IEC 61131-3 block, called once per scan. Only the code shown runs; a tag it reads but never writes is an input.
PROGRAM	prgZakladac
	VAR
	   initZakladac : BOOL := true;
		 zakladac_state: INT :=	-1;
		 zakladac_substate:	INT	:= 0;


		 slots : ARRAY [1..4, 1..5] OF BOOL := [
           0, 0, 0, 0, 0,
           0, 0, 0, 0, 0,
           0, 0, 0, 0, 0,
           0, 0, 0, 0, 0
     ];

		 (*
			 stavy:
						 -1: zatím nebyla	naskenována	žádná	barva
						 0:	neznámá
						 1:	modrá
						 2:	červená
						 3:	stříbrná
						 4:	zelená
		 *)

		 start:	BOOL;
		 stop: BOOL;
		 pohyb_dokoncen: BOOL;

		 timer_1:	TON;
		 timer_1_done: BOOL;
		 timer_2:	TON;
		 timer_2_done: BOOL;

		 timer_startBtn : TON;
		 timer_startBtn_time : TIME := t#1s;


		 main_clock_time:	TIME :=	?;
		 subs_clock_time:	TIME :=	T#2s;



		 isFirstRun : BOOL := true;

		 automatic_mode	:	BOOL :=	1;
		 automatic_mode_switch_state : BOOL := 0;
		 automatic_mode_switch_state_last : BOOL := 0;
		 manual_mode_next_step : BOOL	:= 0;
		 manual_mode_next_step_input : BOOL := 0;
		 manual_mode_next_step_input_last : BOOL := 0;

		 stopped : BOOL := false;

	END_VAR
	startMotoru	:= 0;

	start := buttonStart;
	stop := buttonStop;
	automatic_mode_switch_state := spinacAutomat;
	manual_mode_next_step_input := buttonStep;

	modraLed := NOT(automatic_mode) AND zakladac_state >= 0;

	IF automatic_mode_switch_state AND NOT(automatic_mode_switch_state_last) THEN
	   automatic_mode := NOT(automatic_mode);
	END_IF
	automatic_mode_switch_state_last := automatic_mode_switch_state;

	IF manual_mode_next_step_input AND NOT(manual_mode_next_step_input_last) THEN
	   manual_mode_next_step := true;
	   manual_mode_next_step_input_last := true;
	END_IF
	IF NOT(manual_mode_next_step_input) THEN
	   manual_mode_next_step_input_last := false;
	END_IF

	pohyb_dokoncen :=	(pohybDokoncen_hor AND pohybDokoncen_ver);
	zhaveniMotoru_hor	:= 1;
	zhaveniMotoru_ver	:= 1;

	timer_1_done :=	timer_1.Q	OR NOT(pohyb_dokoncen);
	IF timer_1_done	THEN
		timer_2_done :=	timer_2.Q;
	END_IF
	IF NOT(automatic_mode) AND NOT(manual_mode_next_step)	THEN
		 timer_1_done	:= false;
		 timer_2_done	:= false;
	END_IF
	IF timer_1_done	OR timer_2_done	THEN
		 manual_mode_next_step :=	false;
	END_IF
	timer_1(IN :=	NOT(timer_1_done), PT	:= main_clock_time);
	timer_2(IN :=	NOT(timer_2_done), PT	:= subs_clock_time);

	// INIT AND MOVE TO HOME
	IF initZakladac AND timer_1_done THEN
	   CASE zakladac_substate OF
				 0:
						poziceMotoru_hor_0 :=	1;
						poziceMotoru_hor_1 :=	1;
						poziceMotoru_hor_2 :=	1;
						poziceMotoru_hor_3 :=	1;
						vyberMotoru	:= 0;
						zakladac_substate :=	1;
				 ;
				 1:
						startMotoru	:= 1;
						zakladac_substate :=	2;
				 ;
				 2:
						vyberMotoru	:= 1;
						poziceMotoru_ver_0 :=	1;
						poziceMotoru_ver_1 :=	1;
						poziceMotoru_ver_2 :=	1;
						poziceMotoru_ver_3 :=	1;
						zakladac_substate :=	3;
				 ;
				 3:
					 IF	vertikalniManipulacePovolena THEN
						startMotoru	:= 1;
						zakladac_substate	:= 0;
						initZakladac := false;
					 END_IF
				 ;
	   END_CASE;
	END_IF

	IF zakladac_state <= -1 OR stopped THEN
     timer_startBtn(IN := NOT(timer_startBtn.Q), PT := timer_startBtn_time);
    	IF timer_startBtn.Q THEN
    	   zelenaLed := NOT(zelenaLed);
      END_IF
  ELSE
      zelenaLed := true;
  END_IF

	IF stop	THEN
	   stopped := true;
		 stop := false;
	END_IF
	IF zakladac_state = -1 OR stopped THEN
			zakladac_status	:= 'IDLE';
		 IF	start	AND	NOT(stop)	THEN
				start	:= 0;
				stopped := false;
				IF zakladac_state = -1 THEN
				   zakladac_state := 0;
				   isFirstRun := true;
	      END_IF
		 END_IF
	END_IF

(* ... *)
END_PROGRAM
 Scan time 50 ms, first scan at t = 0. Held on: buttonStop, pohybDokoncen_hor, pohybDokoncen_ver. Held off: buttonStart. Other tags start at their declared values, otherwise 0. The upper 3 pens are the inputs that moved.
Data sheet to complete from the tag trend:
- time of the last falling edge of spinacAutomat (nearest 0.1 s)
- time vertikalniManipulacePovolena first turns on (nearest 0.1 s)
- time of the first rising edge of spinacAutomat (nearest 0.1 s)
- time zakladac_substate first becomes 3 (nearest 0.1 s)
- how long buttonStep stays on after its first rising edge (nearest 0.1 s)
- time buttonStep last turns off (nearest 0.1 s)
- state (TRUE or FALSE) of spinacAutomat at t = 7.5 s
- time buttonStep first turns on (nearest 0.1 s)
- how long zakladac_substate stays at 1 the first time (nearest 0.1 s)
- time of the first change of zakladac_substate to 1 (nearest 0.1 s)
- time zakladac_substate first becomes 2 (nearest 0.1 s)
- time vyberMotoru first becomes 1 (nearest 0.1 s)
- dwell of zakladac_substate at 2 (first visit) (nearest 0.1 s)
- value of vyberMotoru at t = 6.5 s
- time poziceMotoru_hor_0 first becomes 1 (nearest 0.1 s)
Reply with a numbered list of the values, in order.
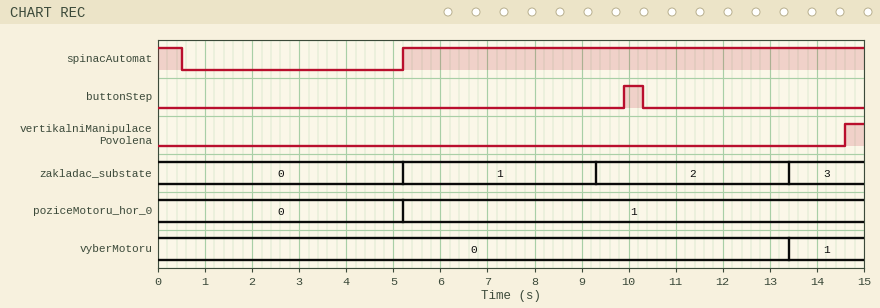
1. 0.5 s
2. 14.6 s
3. 5.2 s
4. 13.4 s
5. 0.4 s
6. 10.3 s
7. TRUE
8. 9.9 s
9. 4.1 s
10. 5.2 s
11. 9.3 s
12. 13.4 s
13. 4.1 s
14. 0
15. 5.2 s
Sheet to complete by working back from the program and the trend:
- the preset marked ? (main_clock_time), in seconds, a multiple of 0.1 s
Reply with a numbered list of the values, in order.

1. 4.0 s
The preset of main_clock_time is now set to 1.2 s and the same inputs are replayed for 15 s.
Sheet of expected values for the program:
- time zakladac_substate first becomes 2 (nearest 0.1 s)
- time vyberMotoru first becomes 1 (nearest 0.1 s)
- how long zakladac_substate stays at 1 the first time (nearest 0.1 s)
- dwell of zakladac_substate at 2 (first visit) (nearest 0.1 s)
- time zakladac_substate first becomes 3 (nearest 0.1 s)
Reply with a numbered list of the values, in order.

1. 6.5 s
2. 7.8 s
3. 1.3 s
4. 1.3 s
5. 7.8 s
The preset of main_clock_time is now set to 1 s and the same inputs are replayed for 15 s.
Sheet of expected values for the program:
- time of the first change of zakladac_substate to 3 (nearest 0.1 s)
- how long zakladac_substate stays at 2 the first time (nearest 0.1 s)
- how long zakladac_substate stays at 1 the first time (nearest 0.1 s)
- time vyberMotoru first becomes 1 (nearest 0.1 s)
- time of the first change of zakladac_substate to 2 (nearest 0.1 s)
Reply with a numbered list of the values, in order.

1. 7.4 s
2. 1.1 s
3. 1.1 s
4. 7.4 s
5. 6.3 s
